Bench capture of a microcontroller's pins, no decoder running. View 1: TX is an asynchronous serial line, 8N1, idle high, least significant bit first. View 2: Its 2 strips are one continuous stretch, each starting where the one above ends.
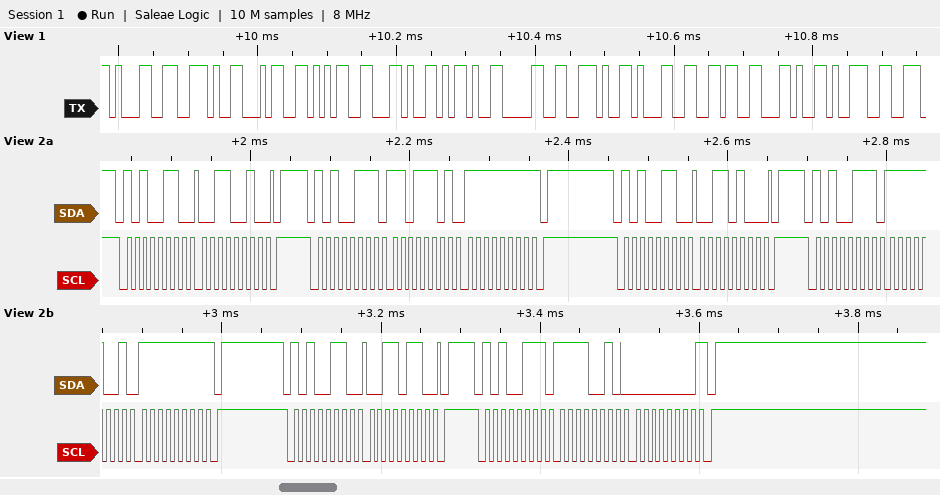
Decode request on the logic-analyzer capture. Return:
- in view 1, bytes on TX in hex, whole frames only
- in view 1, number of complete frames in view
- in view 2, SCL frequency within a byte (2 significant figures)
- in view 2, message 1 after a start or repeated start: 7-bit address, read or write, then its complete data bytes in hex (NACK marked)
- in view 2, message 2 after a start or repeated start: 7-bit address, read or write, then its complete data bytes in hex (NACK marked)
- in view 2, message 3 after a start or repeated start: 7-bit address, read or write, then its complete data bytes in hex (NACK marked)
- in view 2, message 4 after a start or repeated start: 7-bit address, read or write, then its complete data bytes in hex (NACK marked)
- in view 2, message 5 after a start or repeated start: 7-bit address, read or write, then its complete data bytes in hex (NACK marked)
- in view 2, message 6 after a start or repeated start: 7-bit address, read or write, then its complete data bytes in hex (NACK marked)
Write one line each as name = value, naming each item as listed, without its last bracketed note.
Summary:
in view 1, bytes on TX in hex, whole frames only = 31 2E 34 35 2C 2D 30 2E 31 36 2C 39
in view 1, number of complete frames in view = 12
in view 2, SCL frequency within a byte = 100 kHz
in view 2, message 1 after a start or repeated start: 7-bit address, read or write, then its complete data bytes in hex = 0x53 write: 32
in view 2, message 2 after a start or repeated start: 7-bit address, read or write, then its complete data bytes in hex = 0x53 read: DD FF NACK
in view 2, message 3 after a start or repeated start: 7-bit address, read or write, then its complete data bytes in hex = 0x53 write: 34
in view 2, message 4 after a start or repeated start: 7-bit address, read or write, then its complete data bytes in hex = 0x53 read: F9 FF NACK
in view 2, message 5 after a start or repeated start: 7-bit address, read or write, then its complete data bytes in hex = 0x53 write: 36
in view 2, message 6 after a start or repeated start: 7-bit address, read or write, then its complete data bytes in hex = 0x53 read: F2 00 NACK
